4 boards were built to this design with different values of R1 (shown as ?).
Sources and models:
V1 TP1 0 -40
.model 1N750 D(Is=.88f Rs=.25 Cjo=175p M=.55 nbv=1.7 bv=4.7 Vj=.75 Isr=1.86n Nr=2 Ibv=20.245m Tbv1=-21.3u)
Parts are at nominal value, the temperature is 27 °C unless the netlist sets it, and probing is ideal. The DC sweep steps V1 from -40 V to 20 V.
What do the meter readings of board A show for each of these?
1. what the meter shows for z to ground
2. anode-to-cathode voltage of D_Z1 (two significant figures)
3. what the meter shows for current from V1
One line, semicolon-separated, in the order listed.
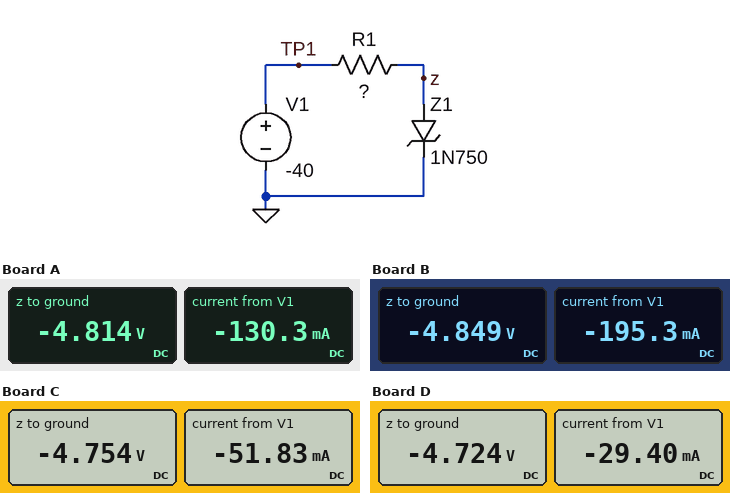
-4.814 V; -4.8 V; -130.3 mA
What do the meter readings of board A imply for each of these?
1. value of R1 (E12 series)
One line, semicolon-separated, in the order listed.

270 Ω
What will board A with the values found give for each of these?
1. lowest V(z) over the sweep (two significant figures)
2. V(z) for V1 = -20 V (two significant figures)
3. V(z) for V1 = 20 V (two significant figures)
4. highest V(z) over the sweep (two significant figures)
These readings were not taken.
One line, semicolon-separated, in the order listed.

-4.8 V; -4.8 V; 840 mV; 840 mV
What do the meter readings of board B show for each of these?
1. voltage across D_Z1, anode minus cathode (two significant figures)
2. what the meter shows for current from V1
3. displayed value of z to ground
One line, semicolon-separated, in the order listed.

-4.8 V; -195.3 mA; -4.849 V
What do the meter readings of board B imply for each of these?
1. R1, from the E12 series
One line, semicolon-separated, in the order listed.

180 Ω
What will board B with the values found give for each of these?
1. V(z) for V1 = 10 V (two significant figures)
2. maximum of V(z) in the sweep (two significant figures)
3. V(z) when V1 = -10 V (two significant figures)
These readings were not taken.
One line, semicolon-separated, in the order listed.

830 mV; 860 mV; -4.7 V
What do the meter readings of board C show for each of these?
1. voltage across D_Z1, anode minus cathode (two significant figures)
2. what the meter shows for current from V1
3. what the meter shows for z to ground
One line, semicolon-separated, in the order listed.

-4.8 V; -51.83 mA; -4.754 V
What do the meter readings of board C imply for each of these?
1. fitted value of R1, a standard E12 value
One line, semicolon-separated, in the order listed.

680 Ω
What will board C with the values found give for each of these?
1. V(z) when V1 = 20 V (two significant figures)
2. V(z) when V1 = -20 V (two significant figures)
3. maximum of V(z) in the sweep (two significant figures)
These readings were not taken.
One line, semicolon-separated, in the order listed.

810 mV; -4.7 V; 810 mV
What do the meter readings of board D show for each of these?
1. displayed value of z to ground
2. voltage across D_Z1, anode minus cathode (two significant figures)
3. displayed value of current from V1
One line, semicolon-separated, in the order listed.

-4.724 V; -4.7 V; -29.40 mA
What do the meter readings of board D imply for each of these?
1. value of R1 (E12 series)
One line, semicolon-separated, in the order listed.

1.2 kΩ
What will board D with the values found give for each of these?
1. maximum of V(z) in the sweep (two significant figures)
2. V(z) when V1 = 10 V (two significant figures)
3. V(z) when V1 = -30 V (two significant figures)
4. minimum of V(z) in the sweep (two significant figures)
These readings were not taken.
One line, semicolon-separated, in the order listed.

790 mV; 770 mV; -4.7 V; -4.7 V
